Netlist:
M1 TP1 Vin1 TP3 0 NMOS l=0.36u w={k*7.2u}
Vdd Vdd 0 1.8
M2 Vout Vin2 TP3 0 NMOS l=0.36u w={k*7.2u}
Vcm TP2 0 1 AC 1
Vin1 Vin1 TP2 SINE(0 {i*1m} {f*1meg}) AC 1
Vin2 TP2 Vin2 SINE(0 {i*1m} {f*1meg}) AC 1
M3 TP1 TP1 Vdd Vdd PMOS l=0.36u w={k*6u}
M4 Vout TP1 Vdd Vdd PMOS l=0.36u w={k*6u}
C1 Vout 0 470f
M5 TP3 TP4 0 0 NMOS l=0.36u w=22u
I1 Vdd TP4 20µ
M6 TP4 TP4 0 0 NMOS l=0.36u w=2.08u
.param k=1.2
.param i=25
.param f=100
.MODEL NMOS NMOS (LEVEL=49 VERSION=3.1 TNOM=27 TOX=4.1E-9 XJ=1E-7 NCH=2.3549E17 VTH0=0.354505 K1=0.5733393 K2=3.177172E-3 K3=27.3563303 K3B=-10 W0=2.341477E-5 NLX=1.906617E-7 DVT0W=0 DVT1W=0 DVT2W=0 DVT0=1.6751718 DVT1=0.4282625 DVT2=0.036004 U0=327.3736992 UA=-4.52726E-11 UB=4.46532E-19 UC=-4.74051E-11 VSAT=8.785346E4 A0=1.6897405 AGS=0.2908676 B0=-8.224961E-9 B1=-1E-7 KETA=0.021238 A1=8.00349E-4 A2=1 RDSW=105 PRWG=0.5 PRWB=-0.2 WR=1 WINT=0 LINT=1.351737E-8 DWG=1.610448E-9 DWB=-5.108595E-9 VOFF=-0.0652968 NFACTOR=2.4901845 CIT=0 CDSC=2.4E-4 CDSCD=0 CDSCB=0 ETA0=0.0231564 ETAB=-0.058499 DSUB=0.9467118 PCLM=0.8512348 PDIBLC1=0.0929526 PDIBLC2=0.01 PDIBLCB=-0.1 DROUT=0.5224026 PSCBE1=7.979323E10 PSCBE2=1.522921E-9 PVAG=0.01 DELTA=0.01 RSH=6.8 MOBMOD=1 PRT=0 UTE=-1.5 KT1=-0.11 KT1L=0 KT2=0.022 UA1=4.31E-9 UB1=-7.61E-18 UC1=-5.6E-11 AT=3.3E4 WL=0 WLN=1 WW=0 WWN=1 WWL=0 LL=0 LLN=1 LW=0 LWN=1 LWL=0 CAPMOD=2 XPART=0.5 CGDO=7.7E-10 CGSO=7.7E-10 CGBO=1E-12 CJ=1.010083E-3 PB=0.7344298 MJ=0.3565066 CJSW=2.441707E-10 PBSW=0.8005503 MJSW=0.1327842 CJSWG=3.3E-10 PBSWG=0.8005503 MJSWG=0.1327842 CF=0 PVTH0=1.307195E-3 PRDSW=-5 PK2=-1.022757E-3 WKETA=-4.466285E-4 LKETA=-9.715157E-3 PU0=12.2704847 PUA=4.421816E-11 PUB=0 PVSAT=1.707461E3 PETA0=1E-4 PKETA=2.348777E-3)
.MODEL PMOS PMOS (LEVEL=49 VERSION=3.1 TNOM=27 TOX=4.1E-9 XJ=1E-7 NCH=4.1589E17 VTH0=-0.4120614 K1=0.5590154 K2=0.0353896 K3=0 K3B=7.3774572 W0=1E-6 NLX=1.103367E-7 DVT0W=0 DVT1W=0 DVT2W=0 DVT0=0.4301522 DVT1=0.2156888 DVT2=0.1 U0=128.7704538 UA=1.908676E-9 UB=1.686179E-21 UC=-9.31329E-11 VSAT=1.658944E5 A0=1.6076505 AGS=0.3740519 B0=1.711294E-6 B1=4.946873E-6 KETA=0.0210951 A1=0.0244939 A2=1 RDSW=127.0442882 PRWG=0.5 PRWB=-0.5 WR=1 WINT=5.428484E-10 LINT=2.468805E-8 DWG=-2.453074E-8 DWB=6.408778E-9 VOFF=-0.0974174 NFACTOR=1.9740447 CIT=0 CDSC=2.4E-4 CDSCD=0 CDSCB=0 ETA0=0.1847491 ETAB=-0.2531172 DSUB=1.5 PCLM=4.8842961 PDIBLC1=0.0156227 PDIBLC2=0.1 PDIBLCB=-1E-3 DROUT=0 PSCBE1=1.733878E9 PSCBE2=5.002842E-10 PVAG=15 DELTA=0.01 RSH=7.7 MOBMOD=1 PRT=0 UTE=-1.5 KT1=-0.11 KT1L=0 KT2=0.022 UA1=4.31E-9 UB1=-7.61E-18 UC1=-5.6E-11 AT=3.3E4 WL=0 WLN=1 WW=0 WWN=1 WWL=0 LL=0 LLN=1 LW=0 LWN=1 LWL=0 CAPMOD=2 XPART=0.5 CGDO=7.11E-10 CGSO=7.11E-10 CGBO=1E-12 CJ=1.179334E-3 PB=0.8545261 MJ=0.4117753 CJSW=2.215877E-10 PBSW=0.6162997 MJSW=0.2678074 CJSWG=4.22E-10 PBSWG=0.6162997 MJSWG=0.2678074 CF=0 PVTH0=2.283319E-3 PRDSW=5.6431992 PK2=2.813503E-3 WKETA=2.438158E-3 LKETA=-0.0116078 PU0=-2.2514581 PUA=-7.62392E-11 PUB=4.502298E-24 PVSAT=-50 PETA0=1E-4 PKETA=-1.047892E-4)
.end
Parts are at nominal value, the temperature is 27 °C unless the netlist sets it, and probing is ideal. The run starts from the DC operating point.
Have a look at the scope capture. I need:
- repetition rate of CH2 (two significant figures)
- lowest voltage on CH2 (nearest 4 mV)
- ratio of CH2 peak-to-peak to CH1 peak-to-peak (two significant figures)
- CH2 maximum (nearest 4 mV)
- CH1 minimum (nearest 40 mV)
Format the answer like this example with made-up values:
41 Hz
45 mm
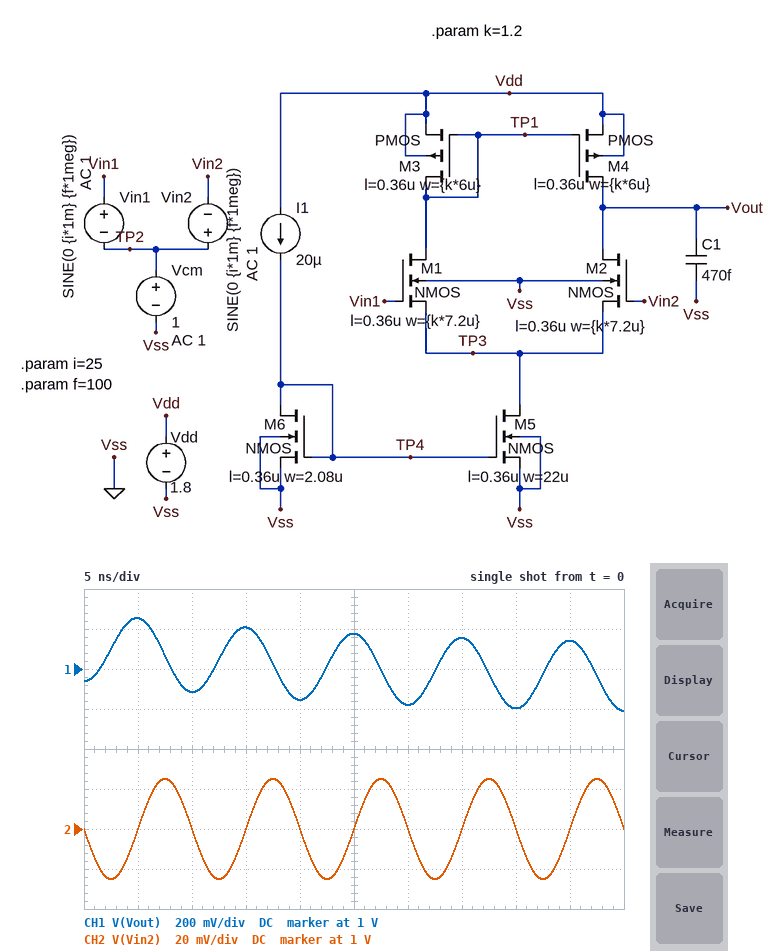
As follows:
100 MHz
976 mV
0.11
1.024 V
800 mV
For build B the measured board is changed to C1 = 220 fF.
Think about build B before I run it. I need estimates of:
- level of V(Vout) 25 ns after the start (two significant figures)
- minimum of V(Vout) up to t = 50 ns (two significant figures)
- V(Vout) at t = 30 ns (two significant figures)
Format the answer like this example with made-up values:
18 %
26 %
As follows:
1.3 V
600 mV
620 mV
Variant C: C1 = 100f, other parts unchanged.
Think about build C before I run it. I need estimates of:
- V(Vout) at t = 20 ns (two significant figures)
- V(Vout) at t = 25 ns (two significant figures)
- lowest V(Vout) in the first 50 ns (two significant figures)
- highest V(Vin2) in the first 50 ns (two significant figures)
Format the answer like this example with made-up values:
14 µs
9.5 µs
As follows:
440 mV
1.5 V
370 mV
1.0 V
